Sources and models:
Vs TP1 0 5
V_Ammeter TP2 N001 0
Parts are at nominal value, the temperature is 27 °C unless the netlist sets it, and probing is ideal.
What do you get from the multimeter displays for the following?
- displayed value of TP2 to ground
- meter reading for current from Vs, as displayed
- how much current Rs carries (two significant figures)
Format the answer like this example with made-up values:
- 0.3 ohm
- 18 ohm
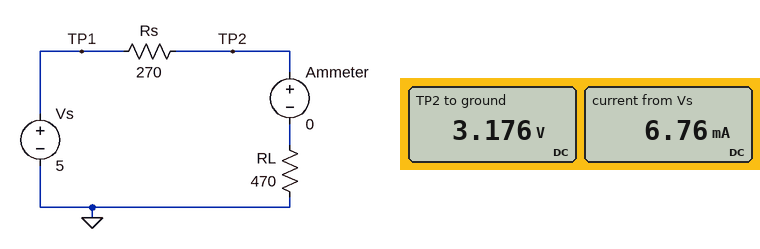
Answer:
- 3.176 V
- 6.76 mA
- 6.8 mA
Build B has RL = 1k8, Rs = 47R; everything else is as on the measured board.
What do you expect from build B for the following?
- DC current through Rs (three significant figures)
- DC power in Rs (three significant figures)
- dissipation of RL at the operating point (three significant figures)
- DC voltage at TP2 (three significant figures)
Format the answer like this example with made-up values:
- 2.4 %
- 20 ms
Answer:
- 2.71 mA
- 344 µW
- 13.2 mW
- 4.87 V
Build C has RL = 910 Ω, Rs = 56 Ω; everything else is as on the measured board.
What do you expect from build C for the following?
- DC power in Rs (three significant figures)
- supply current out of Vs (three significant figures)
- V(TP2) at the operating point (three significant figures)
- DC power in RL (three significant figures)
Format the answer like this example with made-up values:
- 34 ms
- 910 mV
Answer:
- 1.50 mW
- 5.18 mA
- 4.71 V
- 24.4 mW
